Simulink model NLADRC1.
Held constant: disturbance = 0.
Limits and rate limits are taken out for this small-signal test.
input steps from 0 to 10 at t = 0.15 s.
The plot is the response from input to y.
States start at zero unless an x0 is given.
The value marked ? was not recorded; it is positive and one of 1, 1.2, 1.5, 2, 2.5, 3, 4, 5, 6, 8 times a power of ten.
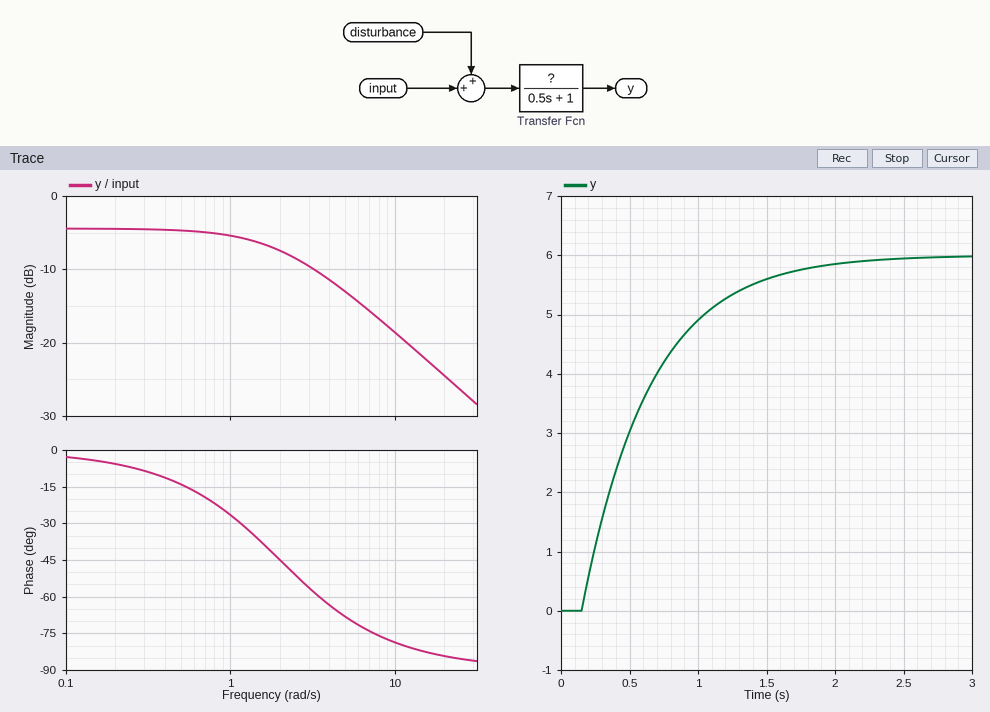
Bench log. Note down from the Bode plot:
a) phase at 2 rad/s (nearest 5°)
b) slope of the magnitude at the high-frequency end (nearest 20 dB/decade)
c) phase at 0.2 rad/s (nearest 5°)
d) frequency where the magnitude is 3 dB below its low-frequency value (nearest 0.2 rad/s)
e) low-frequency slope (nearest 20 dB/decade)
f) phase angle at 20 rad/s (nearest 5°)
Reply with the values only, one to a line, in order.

-45°
-20 dB/decade
-5°
2.0 rad/s
0 dB/decade
-85°
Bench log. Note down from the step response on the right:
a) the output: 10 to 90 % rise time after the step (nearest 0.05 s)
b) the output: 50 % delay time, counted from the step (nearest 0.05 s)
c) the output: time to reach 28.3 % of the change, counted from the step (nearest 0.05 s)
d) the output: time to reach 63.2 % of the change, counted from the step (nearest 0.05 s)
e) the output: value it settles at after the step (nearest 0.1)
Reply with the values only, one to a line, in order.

1.10 s
0.35 s
0.15 s
0.50 s
6.0
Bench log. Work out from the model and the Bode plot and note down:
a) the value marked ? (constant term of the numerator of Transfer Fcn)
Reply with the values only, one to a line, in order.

0.6
